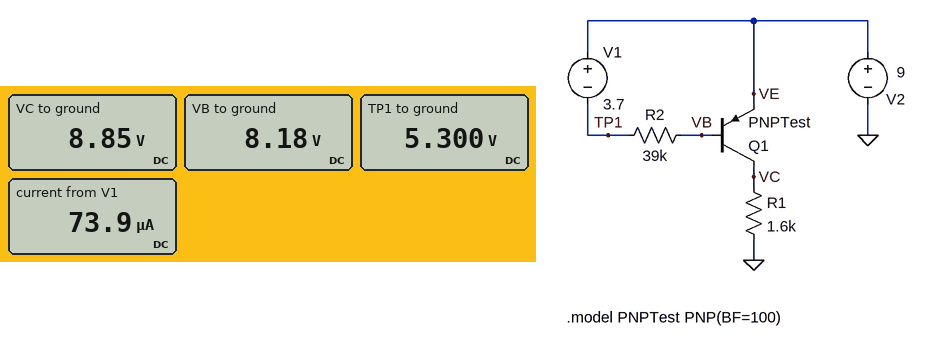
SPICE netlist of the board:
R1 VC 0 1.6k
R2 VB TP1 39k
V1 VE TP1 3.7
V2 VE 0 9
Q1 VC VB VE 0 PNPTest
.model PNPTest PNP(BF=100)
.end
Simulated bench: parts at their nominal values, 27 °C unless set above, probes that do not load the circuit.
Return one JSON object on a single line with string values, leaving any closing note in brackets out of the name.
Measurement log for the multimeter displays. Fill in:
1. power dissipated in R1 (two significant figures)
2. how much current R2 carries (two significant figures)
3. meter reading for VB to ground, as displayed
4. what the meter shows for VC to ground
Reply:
{"power dissipated in R1": "49 mW", "how much current R2 carries": "74 µA", "meter reading for VB to ground, as displayed": "8.18 V", "what the meter shows for VC to ground": "8.85 V"}
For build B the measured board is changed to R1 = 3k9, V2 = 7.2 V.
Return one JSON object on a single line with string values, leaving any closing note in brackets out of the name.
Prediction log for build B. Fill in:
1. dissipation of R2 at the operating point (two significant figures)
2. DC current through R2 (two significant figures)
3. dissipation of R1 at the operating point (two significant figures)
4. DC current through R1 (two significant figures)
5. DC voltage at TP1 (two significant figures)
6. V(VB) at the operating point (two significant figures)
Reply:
{"dissipation of R2 at the operating point": "220 µW", "DC current through R2": "75 µA", "dissipation of R1 at the operating point": "13 mW", "DC current through R1": "1.8 mA", "DC voltage at TP1": "3.5 V", "V(VB) at the operating point": "6.4 V"}
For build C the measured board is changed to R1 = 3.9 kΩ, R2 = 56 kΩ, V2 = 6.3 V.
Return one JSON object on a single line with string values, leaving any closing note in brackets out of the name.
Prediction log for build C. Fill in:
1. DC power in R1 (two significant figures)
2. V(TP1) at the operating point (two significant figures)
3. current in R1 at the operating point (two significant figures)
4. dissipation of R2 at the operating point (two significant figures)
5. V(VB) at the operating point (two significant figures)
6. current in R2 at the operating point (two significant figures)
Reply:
{"DC power in R1": "9.9 mW", "V(TP1) at the operating point": "2.6 V", "current in R1 at the operating point": "1.6 mA", "dissipation of R2 at the operating point": "150 µW", "V(VB) at the operating point": "5.5 V", "current in R2 at the operating point": "52 µA"}
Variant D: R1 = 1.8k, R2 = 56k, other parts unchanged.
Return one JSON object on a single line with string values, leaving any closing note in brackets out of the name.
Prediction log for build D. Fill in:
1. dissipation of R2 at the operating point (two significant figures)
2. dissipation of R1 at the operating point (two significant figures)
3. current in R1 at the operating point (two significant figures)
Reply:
{"dissipation of R2 at the operating point": "150 µW", "dissipation of R1 at the operating point": "43 mW", "current in R1 at the operating point": "4.9 mA"}
